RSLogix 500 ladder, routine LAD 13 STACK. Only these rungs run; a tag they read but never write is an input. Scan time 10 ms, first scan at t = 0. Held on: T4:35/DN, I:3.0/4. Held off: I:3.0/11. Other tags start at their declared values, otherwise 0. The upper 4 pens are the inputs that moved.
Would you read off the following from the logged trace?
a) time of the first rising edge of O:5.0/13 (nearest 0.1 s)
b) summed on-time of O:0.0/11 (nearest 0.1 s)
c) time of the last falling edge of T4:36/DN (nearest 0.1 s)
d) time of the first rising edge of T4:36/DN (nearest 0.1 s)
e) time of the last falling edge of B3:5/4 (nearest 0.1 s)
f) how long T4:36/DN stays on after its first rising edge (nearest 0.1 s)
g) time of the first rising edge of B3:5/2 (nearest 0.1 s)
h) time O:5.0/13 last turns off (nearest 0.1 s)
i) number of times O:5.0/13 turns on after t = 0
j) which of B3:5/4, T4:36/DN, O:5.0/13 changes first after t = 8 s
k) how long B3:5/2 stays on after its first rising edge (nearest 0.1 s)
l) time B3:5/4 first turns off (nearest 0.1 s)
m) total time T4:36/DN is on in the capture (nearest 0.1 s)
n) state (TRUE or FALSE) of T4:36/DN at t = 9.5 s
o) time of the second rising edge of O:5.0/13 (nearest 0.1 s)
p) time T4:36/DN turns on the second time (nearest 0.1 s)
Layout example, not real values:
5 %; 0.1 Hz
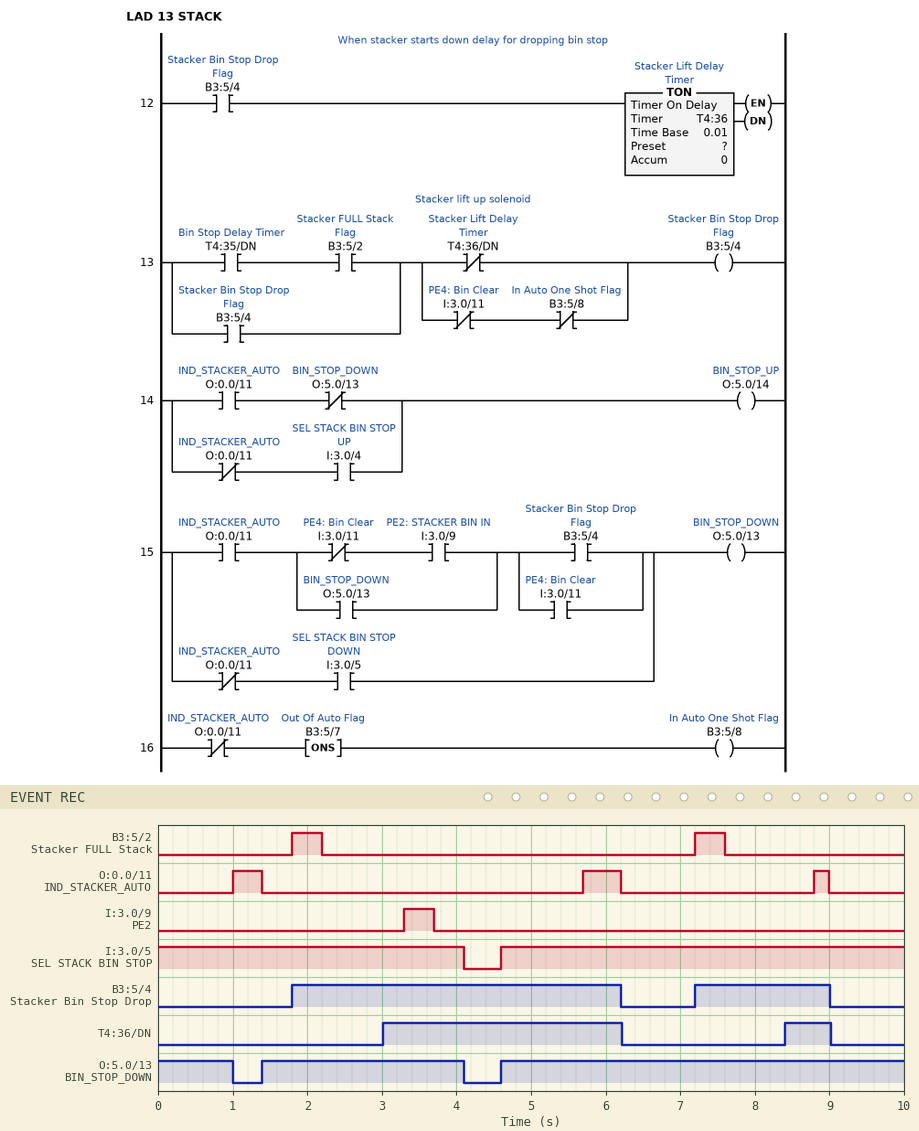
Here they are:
1.4 s; 1.1 s; 9.0 s; 3.0 s; 9.0 s; 3.2 s; 1.8 s; 4.1 s; 2; T4:36/DN; 0.4 s; 6.2 s; 3.8 s; FALSE; 4.6 s; 8.4 s
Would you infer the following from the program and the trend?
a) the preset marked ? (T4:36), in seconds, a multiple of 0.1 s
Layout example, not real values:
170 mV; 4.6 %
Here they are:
1.2 s
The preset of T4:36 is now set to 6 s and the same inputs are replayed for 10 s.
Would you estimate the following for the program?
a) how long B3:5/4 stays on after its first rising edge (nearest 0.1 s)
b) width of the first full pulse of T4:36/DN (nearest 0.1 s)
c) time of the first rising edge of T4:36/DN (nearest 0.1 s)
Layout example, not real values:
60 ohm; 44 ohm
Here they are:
7.2 s; 1.2 s; 7.8 s
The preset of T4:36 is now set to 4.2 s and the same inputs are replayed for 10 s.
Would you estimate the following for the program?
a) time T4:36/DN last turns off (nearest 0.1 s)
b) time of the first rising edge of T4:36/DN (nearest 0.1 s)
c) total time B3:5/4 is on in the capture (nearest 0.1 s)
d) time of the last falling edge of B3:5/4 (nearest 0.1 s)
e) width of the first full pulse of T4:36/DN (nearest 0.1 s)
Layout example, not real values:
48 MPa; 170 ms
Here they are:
6.2 s; 6.0 s; 7.2 s; 6.2 s; 0.2 s
